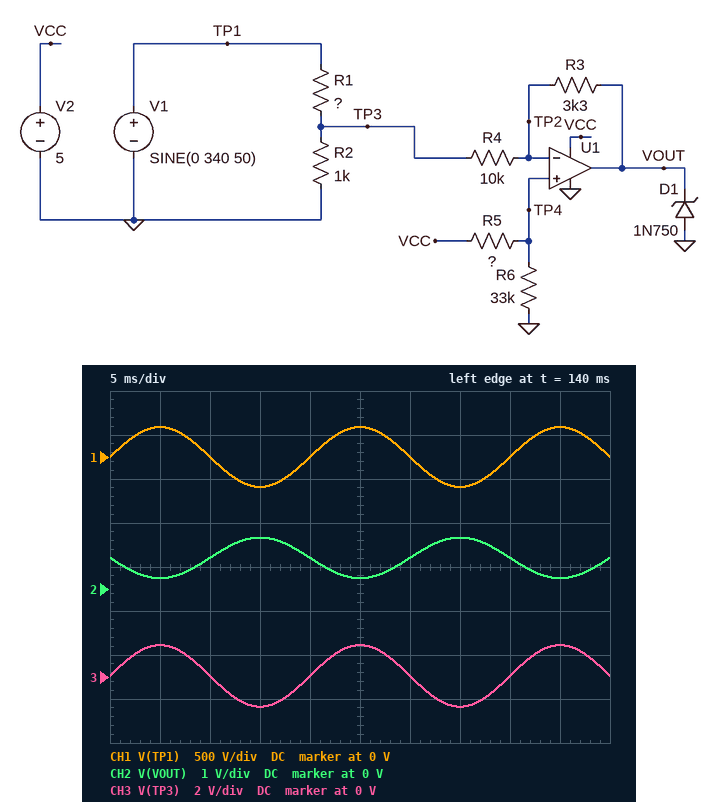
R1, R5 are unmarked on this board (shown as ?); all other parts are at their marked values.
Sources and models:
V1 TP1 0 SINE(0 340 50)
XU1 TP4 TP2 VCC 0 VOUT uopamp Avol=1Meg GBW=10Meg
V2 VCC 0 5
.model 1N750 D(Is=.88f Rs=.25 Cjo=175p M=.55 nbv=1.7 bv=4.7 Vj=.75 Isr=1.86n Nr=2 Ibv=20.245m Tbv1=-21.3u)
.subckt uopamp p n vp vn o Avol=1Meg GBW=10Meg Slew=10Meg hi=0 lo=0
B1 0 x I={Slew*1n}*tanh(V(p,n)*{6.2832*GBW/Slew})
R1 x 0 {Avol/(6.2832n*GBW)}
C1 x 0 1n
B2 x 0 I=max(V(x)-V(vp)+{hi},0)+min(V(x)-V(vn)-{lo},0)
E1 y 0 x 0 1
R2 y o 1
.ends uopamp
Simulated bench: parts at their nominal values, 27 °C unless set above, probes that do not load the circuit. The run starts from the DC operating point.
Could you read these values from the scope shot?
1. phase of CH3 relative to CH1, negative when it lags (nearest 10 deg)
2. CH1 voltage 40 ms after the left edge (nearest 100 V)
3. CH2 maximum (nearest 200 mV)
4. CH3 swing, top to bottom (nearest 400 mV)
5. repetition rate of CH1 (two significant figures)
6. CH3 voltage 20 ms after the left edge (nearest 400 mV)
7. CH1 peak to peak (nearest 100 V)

0 deg
0 V
1.2 V
2.8 V
50 Hz
0 V
700 V
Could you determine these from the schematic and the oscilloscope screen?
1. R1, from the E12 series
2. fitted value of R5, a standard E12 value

220 kΩ
270 kΩ
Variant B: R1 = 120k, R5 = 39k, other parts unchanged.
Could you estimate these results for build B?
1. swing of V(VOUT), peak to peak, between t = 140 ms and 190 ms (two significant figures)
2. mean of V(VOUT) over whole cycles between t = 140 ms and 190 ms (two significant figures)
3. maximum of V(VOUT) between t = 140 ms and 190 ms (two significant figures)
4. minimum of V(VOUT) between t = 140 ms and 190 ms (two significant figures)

1.7 V
3.0 V
3.8 V
2.1 V
